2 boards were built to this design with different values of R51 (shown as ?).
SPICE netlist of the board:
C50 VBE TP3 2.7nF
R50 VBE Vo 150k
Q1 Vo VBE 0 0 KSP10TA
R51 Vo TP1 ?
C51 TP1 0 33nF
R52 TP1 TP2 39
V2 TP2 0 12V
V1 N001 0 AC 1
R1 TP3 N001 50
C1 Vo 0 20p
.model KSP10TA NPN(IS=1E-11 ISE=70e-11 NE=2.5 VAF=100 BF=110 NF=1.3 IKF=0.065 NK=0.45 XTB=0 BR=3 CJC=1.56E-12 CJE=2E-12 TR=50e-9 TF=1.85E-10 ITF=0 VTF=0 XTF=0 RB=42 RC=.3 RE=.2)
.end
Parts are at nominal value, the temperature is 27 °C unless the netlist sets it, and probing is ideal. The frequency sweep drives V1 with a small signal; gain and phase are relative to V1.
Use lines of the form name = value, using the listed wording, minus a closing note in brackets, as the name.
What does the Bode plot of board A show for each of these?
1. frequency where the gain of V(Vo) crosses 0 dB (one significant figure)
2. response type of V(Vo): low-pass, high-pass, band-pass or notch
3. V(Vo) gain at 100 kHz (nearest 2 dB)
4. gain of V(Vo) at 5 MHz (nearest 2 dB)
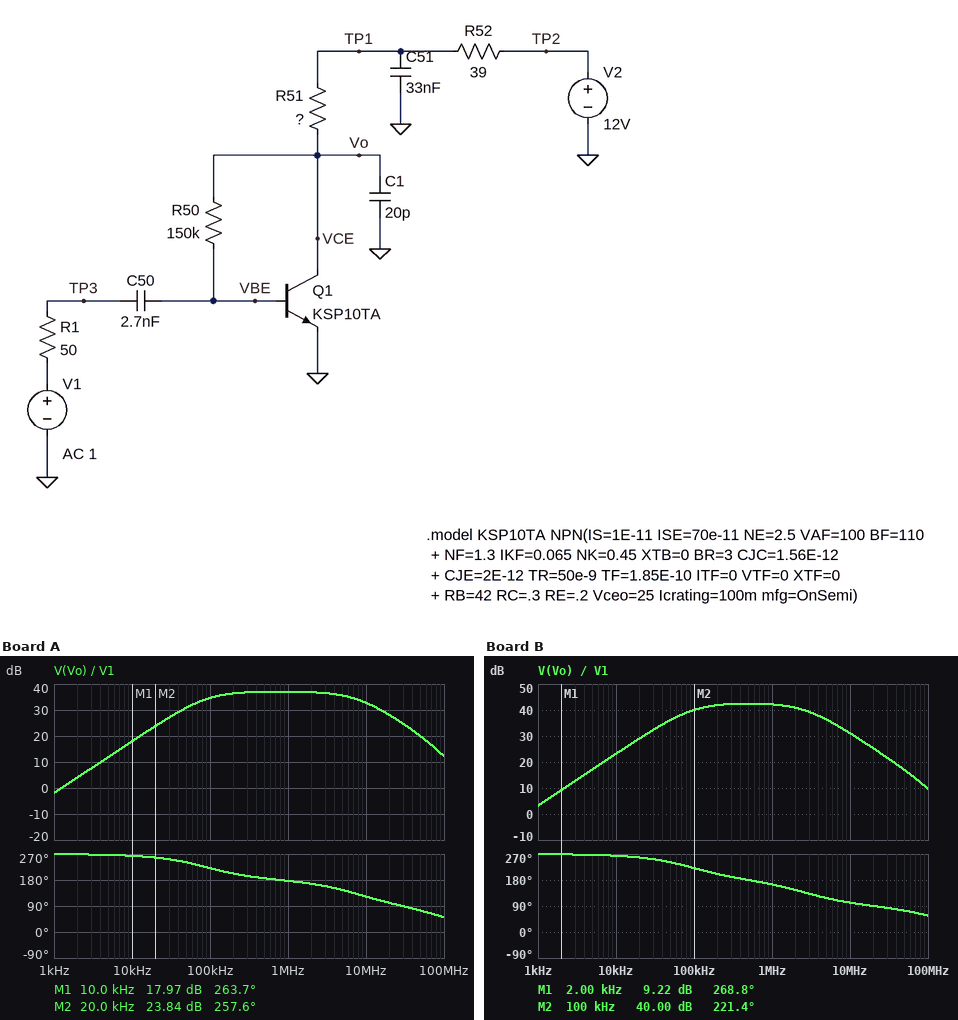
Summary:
frequency where the gain of V(Vo) crosses 0 dB = 1 kHz
response type of V(Vo): low-pass, high-pass, band-pass or notch = band-pass
V(Vo) gain at 100 kHz = 34 dB
gain of V(Vo) at 5 MHz = 36 dB
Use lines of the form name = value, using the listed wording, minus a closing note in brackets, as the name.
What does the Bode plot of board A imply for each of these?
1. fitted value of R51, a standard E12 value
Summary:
fitted value of R51, a standard E12 value = 820 Ω
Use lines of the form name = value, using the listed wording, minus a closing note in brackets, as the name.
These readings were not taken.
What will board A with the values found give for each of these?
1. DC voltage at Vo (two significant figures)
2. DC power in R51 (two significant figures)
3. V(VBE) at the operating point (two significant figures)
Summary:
DC voltage at Vo = 8.7 V
DC power in R51 = 12 mW
V(VBE) at the operating point = 670 mV
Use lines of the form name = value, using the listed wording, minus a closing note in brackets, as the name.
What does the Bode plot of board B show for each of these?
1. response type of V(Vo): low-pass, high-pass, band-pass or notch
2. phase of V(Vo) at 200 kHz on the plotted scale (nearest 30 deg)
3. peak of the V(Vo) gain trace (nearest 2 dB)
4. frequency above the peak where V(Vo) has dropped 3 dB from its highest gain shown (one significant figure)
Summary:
response type of V(Vo): low-pass, high-pass, band-pass or notch = band-pass
phase of V(Vo) at 200 kHz on the plotted scale = 210 deg
peak of the V(Vo) gain trace = 42 dB
frequency above the peak where V(Vo) has dropped 3 dB from its highest gain shown = 3 MHz
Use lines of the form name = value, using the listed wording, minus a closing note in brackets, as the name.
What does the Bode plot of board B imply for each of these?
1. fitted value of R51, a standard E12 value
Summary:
fitted value of R51, a standard E12 value = 2.7 kΩ
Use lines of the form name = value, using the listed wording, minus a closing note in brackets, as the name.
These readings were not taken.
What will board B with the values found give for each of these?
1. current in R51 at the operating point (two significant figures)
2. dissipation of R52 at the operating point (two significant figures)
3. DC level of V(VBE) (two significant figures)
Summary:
current in R51 at the operating point = 2.2 mA
dissipation of R52 at the operating point = 200 µW
DC level of V(VBE) = 650 mV
